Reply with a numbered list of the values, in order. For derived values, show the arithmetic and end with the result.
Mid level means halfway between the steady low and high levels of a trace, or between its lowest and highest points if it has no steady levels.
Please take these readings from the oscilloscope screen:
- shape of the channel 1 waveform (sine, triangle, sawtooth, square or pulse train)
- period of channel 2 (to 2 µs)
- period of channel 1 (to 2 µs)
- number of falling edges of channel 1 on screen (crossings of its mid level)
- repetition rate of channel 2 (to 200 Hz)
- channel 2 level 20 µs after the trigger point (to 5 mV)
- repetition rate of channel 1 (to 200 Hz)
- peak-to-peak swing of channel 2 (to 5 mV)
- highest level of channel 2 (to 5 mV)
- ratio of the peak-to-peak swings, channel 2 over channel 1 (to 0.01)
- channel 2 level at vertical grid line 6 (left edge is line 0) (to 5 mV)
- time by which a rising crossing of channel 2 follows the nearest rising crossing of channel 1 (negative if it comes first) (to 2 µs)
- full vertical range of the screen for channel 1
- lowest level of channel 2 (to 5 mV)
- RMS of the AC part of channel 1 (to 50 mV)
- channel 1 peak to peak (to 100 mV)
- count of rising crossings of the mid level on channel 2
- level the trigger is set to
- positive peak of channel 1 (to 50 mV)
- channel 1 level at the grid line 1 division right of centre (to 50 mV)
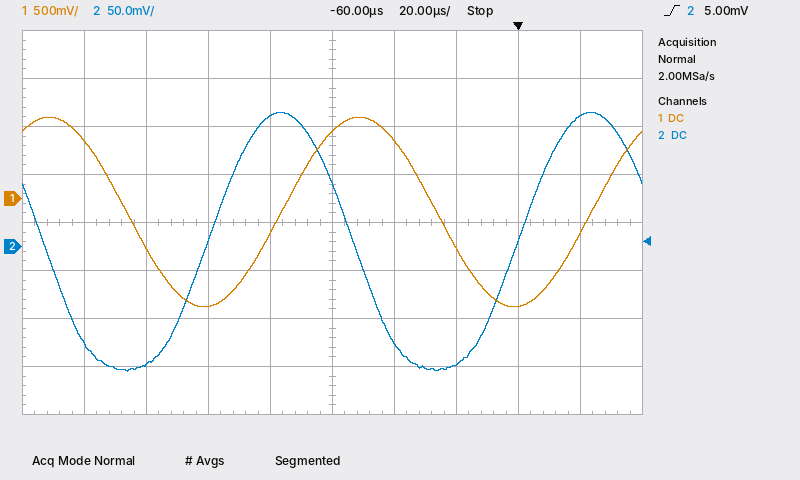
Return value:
1. sine
2. 100 µs
3. 100 µs
4. 2
5. 1 / 100 µs ≈ 10.0 kHz
6. 135 mV
7. 1 / 100 µs ≈ 10.0 kHz
8. 140 mV − (-130 mV) = 270 mV
9. 140 mV
10. 270 mV / 2.00 V ≈ 0.14
11. -100 mV
12. -24 µs
13. 4 V
14. -130 mV
15. 2.00 V / (2√2) ≈ 707 mV, so 700 mV to the nearest 50 mV
16. 2.00 V
17. 2
18. 5.00 mV
19. 850 mV
20. 600 mV
